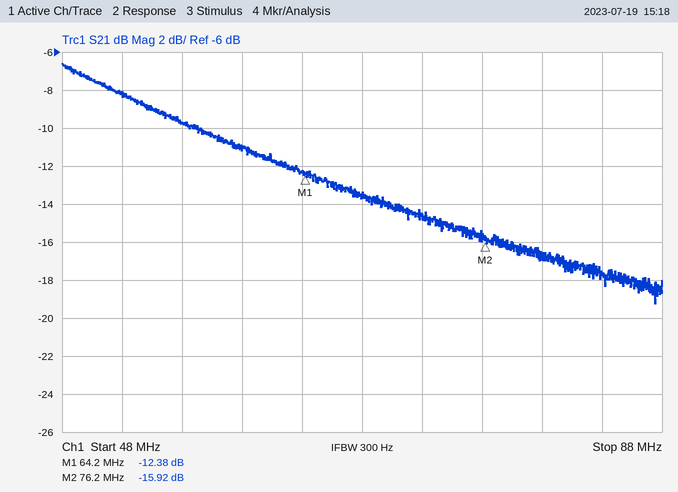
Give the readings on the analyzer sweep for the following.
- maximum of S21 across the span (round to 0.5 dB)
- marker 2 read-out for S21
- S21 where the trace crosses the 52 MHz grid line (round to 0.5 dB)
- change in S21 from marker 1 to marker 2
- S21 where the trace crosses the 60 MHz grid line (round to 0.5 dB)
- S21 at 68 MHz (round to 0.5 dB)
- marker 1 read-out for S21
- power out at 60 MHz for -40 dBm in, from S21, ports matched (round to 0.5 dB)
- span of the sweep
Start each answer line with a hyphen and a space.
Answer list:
- -6.5 dB
- -15.92 dB
- -8.0 dB
- -3.54 dB
- -11.0 dB
- -13.5 dB
- -12.38 dB
- -51.0 dBm
- 40 MHz
